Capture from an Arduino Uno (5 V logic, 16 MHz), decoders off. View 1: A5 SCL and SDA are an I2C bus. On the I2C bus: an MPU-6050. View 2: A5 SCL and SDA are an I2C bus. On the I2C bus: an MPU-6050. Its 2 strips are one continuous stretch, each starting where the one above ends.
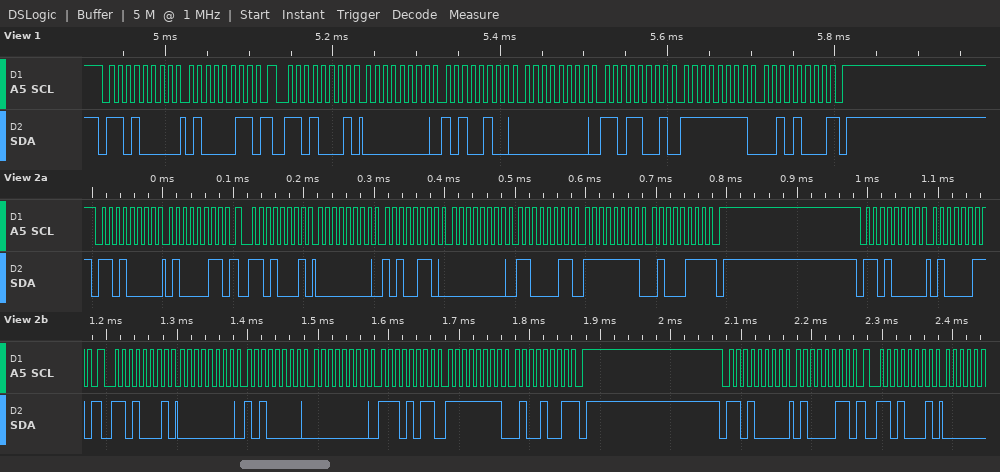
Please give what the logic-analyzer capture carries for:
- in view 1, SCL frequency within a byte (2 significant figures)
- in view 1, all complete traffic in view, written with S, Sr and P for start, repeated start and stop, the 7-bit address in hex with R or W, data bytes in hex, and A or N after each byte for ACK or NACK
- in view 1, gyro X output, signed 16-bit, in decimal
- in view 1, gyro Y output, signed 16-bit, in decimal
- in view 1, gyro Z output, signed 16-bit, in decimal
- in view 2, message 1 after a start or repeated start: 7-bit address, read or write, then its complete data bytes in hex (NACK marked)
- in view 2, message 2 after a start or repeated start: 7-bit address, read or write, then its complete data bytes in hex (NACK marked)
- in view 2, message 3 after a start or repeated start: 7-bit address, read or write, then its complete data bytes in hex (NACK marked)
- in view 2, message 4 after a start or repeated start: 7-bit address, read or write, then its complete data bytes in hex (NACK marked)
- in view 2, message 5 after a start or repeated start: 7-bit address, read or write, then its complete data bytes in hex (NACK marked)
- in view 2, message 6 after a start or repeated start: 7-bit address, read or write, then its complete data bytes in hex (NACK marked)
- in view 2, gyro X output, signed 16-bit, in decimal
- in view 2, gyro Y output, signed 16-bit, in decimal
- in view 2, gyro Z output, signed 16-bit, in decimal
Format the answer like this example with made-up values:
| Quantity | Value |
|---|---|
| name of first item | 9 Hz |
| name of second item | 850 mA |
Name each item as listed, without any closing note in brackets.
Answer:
| Quantity | Value |
|---|---|
| in view 1, SCL frequency within a byte | 100 kHz |
| in view 1, all complete traffic in view, written with S, Sr and P for start, repeated start and stop, the 7-bit address in hex with R or W, data bytes in hex, and A or N after each byte for ACK or NACK | S 68W A 43 A Sr 68R A 00 A A4 A 00 A D9 A FF A 28 N P |
| in view 1, gyro X output, signed 16-bit, in decimal | 164 |
| in view 1, gyro Y output, signed 16-bit, in decimal | 217 |
| in view 1, gyro Z output, signed 16-bit, in decimal | -216 |
| in view 2, message 1 after a start or repeated start: 7-bit address, read or write, then its complete data bytes in hex | 0x68 write: 43 |
| in view 2, message 2 after a start or repeated start: 7-bit address, read or write, then its complete data bytes in hex | 0x68 read: 00 A6 00 C3 FF 47 NACK |
| in view 2, message 3 after a start or repeated start: 7-bit address, read or write, then its complete data bytes in hex | 0x68 write: 43 |
| in view 2, message 4 after a start or repeated start: 7-bit address, read or write, then its complete data bytes in hex | 0x68 read: 00 A0 00 EB FF 49 NACK |
| in view 2, message 5 after a start or repeated start: 7-bit address, read or write, then its complete data bytes in hex | 0x68 write: 43 |
| in view 2, message 6 after a start or repeated start: 7-bit address, read or write, then its complete data bytes in hex | 0x68 read |
| in view 2, gyro X output, signed 16-bit, in decimal | 166 |
| in view 2, gyro Y output, signed 16-bit, in decimal | 195 |
| in view 2, gyro Z output, signed 16-bit, in decimal | -185 |
